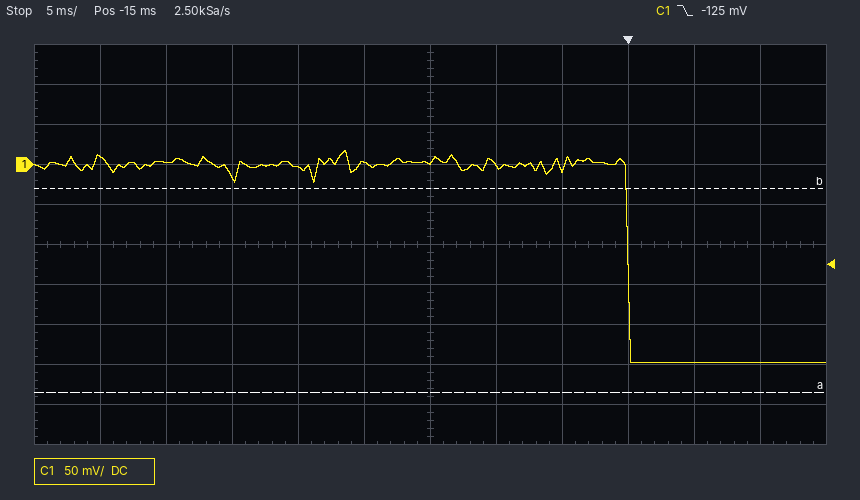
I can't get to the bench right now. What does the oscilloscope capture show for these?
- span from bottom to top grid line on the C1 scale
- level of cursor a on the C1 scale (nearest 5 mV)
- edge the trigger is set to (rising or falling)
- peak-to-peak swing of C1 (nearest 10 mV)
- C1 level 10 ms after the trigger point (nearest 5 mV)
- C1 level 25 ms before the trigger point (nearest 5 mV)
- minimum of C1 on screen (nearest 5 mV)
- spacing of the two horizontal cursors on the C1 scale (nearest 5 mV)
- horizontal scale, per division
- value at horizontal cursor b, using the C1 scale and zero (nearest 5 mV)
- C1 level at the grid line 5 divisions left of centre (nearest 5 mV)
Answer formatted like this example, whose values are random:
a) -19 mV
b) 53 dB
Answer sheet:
a) 500 mV
b) -285 mV
c) falling
d) 270 mV
e) -250 mV
f) -5 mV
g) -250 mV
h) 255 mV
i) 5 ms
j) -30 mV
k) 10 mV
